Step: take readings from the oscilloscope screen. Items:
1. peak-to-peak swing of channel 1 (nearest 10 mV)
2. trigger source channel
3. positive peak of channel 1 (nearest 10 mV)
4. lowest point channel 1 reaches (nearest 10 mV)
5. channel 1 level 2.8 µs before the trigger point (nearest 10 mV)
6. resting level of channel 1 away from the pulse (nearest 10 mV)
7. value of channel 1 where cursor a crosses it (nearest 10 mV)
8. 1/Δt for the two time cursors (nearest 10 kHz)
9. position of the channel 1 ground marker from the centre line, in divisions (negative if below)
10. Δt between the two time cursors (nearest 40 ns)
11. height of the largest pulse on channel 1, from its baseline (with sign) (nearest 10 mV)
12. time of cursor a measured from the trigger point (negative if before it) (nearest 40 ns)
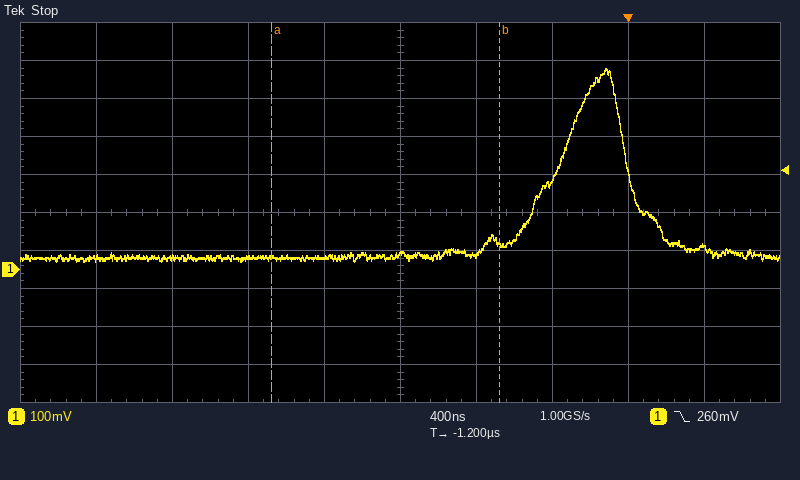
510 mV
channel 1
530 mV
20 mV
30 mV
30 mV
30 mV
830 kHz
-1.5 div
1.20 µs
+500 mV
-1.88 µs
